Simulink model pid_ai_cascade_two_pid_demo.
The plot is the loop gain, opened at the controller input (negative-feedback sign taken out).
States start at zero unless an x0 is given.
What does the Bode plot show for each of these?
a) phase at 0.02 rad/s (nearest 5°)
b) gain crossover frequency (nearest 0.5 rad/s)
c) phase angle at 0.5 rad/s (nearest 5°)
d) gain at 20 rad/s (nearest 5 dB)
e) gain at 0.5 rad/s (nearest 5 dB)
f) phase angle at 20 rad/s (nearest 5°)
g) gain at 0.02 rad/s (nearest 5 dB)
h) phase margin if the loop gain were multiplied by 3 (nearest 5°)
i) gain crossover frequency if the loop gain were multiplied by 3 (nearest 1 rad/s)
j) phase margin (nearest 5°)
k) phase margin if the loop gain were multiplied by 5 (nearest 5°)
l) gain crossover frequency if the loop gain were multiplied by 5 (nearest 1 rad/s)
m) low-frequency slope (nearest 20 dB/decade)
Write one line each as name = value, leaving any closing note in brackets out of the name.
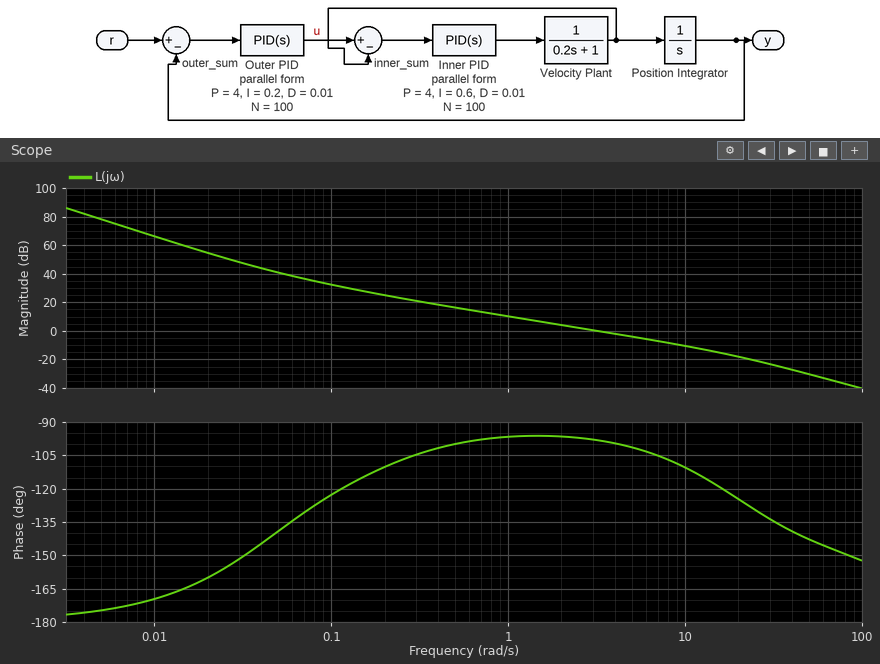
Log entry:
phase at 0.02 rad/s = -160°
gain crossover frequency = 3.0 rad/s
phase angle at 0.5 rad/s = -100°
gain at 20 rad/s = -20 dB
gain at 0.5 rad/s = 15 dB
phase angle at 20 rad/s = -125°
gain at 0.02 rad/s = 55 dB
phase margin if the loop gain were multiplied by 3 = 70°
gain crossover frequency if the loop gain were multiplied by 3 = 9 rad/s
phase margin = 80°
phase margin if the loop gain were multiplied by 5 = 65°
gain crossover frequency if the loop gain were multiplied by 5 = 14 rad/s
low-frequency slope = -40 dB/decade
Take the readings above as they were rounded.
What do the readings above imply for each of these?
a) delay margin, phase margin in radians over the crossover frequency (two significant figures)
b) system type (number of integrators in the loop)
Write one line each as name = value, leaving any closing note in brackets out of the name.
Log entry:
delay margin, phase margin in radians over the crossover frequency = 0.47 s
system type = 2
